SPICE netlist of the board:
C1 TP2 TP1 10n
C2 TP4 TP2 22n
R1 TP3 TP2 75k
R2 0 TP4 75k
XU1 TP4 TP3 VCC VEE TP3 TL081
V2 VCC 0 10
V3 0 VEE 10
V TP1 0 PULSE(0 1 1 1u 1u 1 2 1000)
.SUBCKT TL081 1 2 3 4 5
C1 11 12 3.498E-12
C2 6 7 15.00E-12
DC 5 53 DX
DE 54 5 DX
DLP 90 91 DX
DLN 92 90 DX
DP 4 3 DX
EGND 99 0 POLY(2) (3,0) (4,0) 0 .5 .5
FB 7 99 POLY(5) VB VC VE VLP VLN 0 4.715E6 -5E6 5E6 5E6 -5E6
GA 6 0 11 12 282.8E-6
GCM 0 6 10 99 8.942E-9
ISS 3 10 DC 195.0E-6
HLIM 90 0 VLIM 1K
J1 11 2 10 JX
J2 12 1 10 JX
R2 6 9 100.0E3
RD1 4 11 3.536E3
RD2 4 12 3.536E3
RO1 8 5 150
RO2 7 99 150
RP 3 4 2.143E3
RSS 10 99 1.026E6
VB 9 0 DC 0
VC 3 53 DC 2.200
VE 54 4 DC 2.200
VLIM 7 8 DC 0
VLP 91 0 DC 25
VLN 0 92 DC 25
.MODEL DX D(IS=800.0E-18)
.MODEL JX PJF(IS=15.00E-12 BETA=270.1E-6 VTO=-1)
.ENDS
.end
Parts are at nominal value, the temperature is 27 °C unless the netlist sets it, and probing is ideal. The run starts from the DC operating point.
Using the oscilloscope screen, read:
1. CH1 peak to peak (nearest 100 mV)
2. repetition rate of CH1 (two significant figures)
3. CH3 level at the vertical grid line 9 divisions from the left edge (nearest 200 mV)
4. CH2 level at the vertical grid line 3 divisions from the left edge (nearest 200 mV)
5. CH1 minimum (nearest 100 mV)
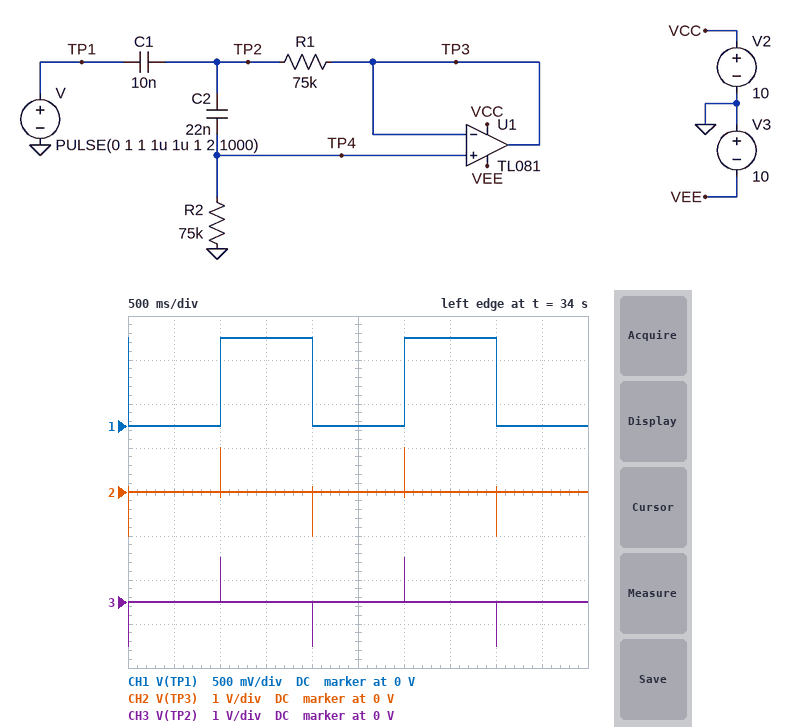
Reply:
1.0 V
500 mHz
0 V
0 V
0 V
